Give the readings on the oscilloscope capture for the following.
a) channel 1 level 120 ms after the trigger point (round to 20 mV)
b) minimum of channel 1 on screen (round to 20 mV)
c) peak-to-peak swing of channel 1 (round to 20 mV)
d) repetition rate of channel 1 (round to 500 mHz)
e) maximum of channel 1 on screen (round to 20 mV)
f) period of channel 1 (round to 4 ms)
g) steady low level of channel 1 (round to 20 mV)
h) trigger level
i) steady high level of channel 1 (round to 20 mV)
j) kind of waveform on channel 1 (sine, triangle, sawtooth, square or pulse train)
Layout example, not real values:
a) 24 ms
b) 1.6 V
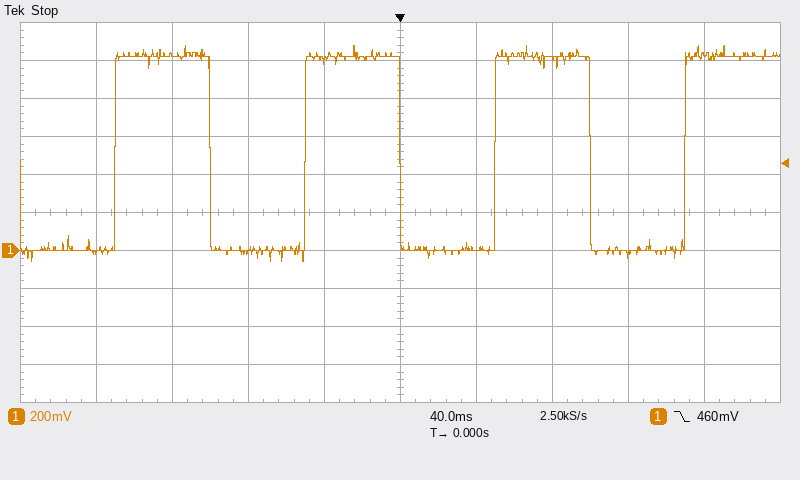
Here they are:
a) -20 mV
b) -60 mV
c) 1.14 V
d) 10.0 Hz
e) 1.08 V
f) 100 ms
g) 0 mV
h) 460 mV
i) 1.02 V
j) square
